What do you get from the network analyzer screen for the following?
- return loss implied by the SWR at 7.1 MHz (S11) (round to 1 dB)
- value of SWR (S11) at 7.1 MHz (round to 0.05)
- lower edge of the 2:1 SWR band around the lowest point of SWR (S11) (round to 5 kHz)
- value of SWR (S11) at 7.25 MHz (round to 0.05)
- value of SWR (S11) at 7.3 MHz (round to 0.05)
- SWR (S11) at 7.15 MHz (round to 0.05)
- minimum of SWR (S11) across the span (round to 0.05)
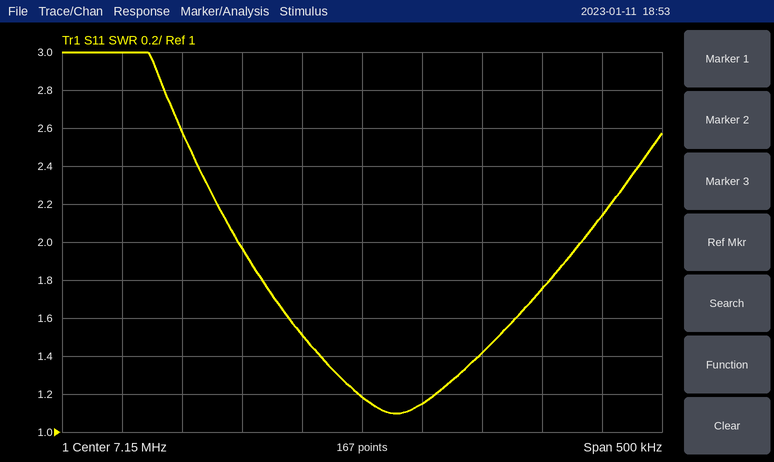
14 dB
1.50
7.045 MHz
1.40
1.75
1.20
1.10
